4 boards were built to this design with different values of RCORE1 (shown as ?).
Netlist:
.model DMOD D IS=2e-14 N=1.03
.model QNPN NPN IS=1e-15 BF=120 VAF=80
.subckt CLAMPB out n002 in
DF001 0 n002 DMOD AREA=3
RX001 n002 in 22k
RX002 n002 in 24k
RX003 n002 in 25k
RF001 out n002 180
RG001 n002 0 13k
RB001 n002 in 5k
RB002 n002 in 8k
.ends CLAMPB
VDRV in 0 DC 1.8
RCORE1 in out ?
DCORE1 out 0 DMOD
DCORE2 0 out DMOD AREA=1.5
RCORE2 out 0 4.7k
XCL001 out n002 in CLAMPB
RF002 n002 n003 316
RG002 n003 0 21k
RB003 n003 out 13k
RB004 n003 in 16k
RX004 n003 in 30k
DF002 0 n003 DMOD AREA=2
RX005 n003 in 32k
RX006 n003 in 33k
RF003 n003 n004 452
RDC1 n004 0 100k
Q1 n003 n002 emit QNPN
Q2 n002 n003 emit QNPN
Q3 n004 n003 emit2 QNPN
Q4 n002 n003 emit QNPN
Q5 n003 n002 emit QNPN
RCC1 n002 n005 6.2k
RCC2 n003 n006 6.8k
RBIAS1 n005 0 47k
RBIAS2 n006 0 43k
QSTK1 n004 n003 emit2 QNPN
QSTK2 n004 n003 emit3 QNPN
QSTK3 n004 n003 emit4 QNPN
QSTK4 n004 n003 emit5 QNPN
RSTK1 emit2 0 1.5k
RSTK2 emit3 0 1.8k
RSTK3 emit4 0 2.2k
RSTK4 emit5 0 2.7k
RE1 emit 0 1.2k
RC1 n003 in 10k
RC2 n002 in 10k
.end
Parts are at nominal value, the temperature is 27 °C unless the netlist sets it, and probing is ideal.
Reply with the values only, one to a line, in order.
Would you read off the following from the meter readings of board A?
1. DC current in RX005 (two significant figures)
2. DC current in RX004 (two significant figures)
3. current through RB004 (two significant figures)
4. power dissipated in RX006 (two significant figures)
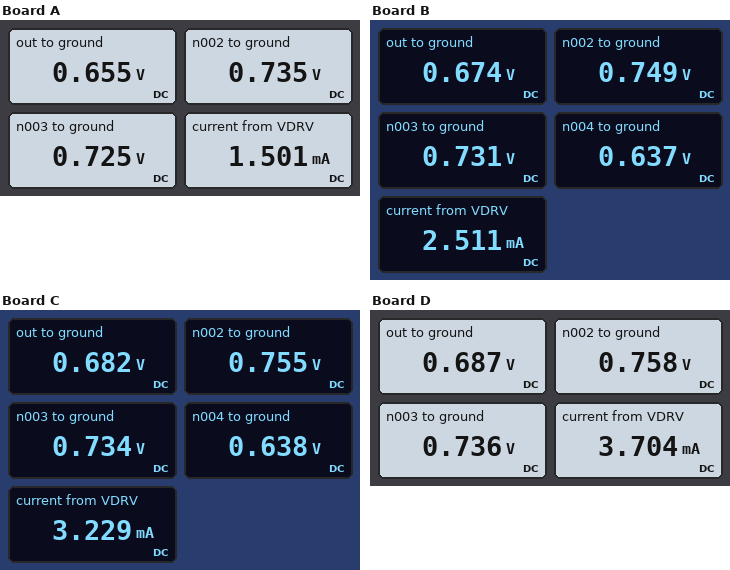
34 µA
36 µA
67 µA
35 µW
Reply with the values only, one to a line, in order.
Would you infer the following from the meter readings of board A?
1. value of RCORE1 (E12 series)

1.8 kΩ
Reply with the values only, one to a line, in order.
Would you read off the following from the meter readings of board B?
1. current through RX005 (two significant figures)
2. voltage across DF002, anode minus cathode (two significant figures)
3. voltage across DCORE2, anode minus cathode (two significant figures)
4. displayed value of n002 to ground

33 µA
-730 mV
-670 mV
0.749 V
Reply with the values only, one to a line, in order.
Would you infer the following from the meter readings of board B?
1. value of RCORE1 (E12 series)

680 Ω
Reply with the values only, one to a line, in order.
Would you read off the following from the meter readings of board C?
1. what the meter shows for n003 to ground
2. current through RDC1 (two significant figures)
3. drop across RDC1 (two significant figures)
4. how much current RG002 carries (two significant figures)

0.734 V
6.4 µA
640 mV
35 µA
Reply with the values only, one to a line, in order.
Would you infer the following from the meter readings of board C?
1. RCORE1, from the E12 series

470 Ω
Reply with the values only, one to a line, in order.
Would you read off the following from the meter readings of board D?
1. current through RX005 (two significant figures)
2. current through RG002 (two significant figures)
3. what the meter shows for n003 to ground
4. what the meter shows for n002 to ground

33 µA
35 µA
0.736 V
0.758 V
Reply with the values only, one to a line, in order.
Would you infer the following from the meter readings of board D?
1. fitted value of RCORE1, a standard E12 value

390 Ω
